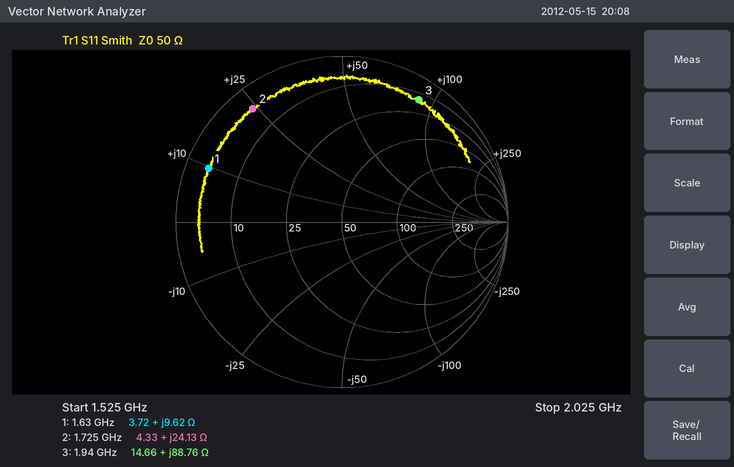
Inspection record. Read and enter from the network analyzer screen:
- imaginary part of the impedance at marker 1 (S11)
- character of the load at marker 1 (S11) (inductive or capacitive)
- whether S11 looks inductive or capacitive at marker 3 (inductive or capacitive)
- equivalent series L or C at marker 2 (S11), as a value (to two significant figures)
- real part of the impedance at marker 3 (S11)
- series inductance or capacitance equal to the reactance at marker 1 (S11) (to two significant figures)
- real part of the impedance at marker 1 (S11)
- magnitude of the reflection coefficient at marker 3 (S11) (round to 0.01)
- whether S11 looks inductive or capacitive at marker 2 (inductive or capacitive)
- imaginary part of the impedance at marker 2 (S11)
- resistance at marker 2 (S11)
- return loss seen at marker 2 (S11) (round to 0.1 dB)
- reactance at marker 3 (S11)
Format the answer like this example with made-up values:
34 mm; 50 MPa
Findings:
+9.62 Ω; inductive; inductive; 2.2 nH; 14.66 Ω; 940 pH; 3.72 Ω; 0.87; inductive; +24.13 Ω; 4.33 Ω; 1.2 dB; +88.76 Ω
